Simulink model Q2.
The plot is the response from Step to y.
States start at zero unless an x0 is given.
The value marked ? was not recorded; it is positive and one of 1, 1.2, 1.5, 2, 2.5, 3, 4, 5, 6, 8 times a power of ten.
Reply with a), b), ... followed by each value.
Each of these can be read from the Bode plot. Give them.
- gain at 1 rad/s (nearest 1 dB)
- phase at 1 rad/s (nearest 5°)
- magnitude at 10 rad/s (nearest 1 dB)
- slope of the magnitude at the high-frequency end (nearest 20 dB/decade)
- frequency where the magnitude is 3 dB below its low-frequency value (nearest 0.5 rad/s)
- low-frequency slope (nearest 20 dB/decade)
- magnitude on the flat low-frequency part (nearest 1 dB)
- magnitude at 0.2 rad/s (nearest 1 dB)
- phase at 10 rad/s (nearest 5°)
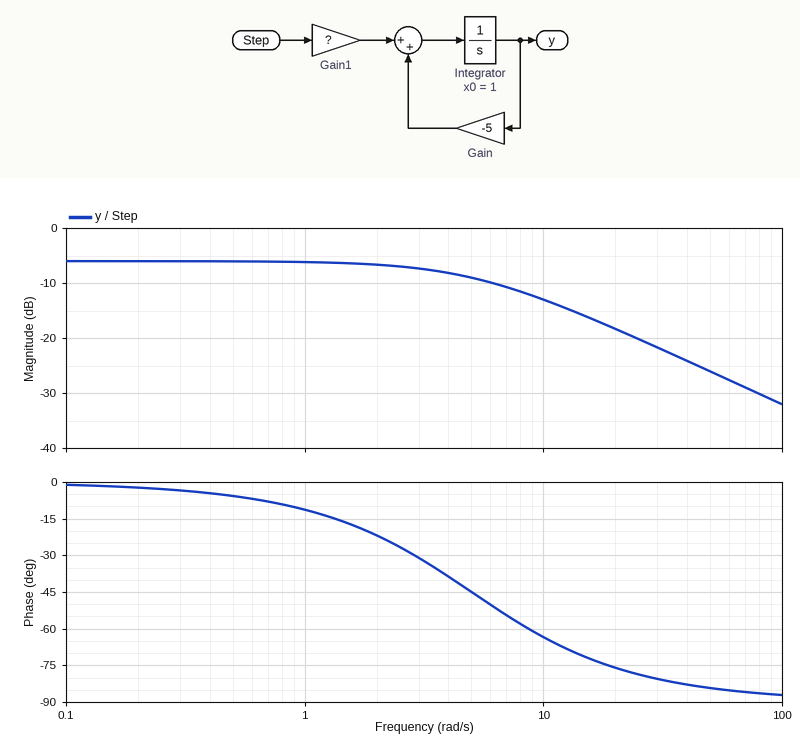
a) -6 dB
b) -10°
c) -13 dB
d) -20 dB/decade
e) 5.0 rad/s
f) 0 dB/decade
g) -6 dB
h) -6 dB
i) -65°
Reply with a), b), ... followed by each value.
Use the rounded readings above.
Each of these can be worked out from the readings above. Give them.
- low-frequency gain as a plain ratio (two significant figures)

a) 0.50
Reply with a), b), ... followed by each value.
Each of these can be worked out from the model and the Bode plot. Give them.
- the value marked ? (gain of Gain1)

a) 2.5
